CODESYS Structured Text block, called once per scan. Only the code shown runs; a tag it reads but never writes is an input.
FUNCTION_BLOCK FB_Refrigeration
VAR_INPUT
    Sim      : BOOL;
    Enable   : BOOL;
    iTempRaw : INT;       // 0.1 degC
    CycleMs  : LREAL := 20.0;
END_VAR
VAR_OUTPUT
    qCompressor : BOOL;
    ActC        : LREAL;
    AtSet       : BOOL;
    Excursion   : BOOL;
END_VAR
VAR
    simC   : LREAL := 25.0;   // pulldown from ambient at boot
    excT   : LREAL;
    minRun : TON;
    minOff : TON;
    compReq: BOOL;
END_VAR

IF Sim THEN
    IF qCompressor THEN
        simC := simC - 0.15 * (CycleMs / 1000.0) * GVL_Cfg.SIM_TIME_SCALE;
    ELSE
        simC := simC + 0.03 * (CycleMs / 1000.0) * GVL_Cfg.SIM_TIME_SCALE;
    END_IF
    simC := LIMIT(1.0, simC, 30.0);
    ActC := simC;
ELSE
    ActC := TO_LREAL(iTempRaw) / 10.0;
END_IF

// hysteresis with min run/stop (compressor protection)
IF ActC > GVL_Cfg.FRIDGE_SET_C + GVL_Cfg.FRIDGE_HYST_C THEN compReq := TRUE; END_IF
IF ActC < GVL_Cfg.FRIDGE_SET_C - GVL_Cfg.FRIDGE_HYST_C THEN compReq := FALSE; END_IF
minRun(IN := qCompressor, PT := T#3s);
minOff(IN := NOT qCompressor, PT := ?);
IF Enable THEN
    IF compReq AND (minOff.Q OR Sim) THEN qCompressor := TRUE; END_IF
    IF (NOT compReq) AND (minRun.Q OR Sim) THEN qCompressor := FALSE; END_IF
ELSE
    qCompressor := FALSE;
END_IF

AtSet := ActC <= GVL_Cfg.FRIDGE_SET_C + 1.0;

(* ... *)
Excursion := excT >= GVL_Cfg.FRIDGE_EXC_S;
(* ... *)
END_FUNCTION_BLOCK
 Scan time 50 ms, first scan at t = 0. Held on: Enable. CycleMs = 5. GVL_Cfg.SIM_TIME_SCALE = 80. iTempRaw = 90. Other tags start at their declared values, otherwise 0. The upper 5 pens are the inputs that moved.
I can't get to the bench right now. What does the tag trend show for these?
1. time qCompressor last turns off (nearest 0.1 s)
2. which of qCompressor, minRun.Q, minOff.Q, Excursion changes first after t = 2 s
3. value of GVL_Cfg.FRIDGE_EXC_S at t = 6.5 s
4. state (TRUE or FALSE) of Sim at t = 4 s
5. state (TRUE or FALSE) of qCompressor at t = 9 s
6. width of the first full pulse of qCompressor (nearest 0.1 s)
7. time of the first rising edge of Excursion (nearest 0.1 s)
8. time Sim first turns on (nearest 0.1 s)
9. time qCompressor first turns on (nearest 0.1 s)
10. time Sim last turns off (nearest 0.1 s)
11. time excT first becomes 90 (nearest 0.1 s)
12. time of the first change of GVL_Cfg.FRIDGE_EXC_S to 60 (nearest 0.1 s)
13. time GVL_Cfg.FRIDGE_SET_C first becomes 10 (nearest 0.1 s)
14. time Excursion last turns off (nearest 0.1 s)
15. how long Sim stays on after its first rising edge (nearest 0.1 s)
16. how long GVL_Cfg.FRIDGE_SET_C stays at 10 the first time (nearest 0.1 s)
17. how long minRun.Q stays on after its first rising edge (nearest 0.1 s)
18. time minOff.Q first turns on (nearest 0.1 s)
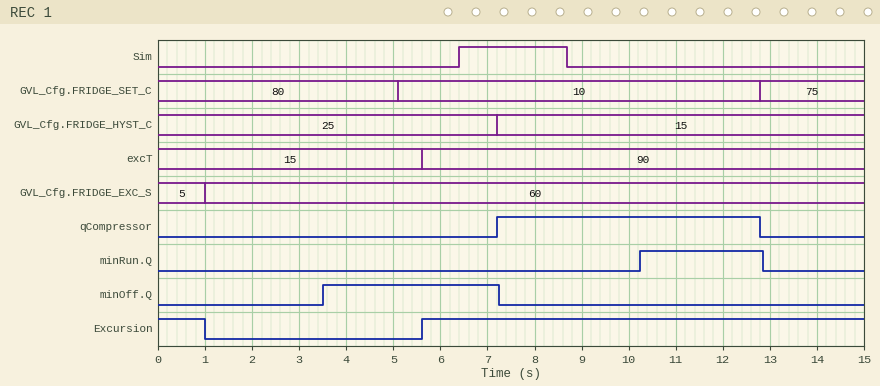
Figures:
12.8 s
minOff.Q
60
FALSE
TRUE
5.6 s
5.6 s
6.4 s
7.2 s
8.7 s
5.6 s
1.0 s
5.1 s
1.0 s
2.3 s
7.7 s
2.6 s
3.5 s
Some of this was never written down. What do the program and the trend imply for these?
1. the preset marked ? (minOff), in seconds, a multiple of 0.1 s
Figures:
3.5 s
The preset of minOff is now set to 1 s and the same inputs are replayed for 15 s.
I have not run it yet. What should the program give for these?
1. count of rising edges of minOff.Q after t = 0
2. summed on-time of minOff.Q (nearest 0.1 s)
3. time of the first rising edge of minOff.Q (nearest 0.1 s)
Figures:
2
7.4 s
1.0 s
